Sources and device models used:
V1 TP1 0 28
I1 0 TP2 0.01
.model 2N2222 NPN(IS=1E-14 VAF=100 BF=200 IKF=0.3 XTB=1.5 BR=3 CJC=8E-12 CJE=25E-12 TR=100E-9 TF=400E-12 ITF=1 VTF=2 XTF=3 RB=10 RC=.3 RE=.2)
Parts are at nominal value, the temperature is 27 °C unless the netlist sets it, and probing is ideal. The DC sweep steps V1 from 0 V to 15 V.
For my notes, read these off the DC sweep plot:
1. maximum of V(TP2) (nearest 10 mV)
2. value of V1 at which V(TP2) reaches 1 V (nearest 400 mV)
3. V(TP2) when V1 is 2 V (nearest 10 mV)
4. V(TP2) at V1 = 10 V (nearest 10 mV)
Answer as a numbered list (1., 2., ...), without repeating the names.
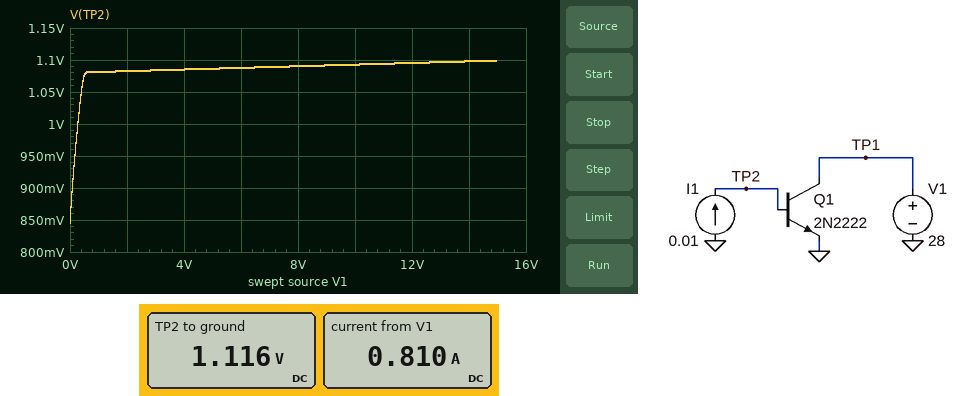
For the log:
1. 1.10 V
2. 400 mV
3. 1.08 V
4. 1.09 V
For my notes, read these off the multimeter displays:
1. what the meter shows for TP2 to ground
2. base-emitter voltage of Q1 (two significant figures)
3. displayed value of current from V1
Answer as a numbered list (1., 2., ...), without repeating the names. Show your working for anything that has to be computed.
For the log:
1. 1.116 V
2. 1.116 V = 1.1 V
3. 0.810 A
